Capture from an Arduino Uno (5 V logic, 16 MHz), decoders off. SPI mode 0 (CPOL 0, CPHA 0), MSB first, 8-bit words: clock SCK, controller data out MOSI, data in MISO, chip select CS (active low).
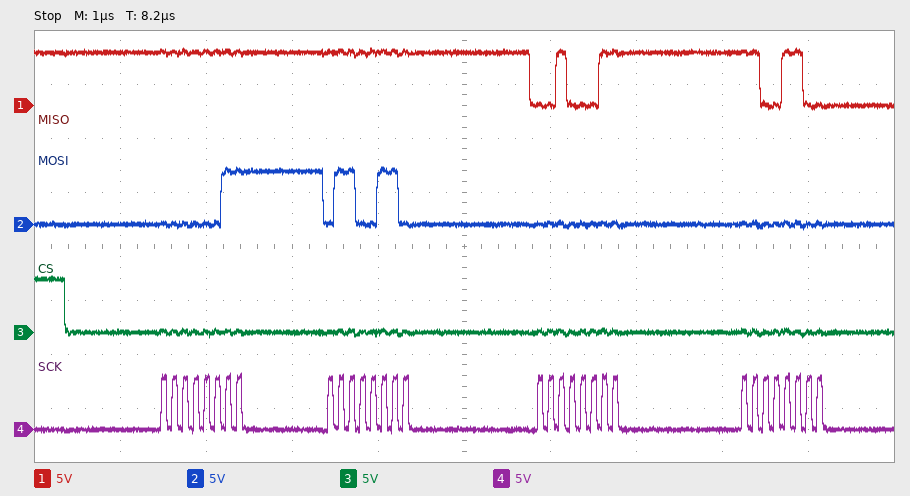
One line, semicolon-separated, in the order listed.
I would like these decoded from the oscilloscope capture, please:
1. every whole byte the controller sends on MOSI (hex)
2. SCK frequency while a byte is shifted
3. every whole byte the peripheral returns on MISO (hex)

03 66 00 00; 8 MHz; FF FF 23 CC
